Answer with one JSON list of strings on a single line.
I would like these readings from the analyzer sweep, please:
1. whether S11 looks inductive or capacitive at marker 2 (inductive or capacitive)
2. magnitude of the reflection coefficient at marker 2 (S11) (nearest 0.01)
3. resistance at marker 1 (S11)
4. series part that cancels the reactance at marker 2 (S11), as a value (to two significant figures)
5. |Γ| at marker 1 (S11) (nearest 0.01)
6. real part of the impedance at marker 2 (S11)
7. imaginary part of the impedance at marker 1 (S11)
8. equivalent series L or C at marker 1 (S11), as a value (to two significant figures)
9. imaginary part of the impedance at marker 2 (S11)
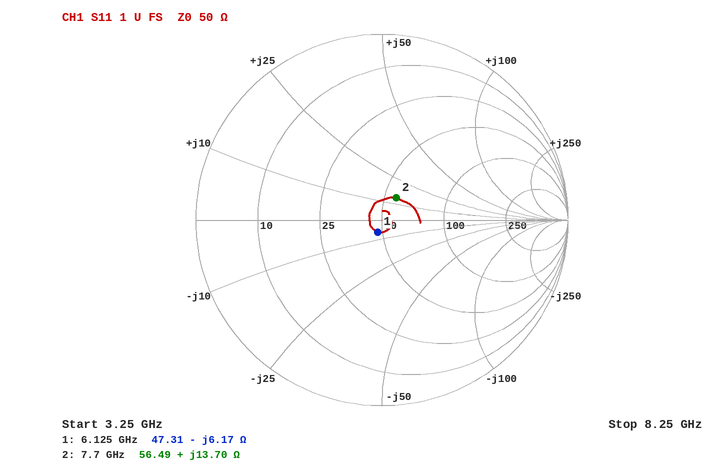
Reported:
["inductive", "0.14", "47.31 Ω", "1.5 pF", "0.07", "56.49 Ω", "-6.17 Ω", "4.2 pF", "+13.70 Ω"]
